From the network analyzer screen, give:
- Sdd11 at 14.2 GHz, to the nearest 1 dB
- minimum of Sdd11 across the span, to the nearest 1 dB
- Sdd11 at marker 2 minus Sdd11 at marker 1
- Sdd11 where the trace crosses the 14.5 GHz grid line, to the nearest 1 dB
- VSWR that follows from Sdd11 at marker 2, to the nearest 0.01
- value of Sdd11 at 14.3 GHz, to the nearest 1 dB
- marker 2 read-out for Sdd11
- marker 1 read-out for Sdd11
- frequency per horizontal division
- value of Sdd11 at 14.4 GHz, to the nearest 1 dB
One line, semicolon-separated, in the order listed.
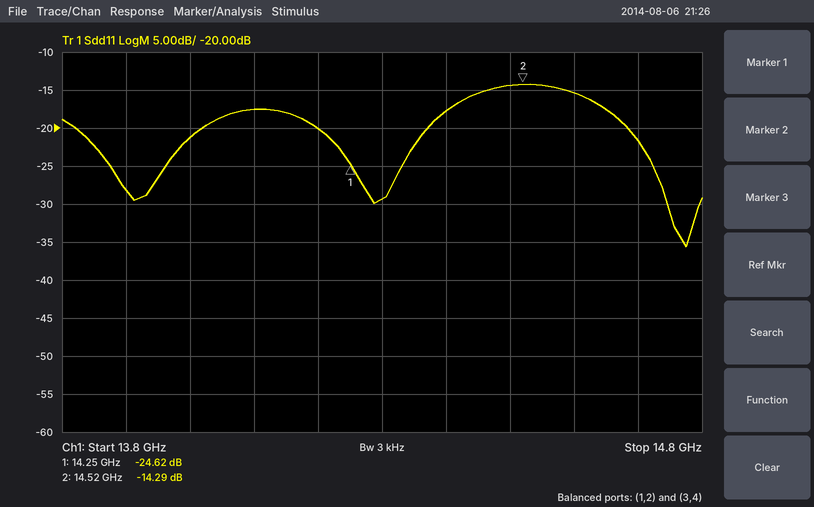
-20 dB; -36 dB; 10.33 dB; -14 dB; 1.48; -29 dB; -14.29 dB; -24.62 dB; 100 MHz; -18 dB
